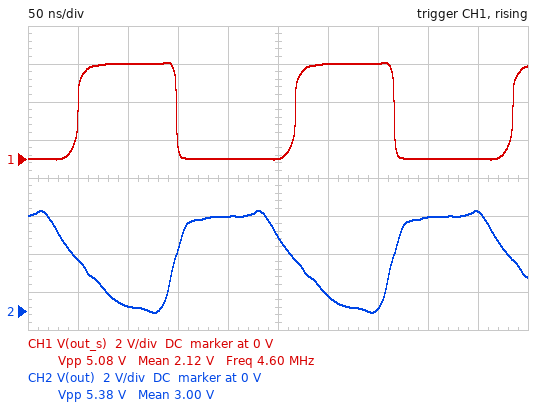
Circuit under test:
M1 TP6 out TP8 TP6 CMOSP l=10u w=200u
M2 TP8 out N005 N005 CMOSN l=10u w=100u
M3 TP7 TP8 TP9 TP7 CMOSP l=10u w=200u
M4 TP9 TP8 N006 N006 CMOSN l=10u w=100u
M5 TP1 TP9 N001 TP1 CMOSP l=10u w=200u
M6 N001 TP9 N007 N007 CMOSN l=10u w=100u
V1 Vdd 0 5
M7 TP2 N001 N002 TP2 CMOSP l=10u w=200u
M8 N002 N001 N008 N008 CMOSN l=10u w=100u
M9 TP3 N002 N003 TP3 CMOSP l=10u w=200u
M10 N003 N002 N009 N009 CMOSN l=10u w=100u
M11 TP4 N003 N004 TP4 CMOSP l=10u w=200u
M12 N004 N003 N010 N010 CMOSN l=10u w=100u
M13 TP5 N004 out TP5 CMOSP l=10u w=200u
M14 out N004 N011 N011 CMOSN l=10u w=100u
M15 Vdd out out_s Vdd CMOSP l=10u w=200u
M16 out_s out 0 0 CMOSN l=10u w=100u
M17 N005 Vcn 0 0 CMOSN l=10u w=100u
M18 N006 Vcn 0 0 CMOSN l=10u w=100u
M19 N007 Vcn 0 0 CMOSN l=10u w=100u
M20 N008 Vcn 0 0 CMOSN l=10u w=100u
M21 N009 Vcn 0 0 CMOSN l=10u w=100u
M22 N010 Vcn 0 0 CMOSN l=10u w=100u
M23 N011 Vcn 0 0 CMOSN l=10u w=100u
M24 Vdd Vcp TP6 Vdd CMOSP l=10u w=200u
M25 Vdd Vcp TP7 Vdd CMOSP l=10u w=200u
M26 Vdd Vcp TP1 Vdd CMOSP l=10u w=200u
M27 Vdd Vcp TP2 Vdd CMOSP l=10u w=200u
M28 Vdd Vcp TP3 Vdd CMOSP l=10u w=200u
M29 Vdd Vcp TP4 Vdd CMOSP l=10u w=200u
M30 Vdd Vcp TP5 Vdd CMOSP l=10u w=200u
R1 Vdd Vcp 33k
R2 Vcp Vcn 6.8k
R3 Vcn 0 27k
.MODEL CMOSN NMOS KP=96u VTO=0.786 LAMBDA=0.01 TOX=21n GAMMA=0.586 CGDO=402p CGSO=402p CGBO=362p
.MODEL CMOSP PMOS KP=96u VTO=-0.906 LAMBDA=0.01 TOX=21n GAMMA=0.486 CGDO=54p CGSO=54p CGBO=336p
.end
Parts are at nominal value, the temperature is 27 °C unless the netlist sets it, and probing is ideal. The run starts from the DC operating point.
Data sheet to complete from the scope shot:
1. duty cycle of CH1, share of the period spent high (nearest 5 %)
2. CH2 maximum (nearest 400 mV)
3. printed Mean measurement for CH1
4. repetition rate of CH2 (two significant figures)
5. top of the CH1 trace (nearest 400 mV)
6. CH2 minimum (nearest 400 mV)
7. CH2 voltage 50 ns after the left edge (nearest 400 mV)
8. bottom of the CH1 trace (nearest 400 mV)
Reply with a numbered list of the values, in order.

1. 45 %
2. 5.2 V
3. 2.12 V
4. 4.6 MHz
5. 5.2 V
6. 0 V
7. 2.8 V
8. 0 V
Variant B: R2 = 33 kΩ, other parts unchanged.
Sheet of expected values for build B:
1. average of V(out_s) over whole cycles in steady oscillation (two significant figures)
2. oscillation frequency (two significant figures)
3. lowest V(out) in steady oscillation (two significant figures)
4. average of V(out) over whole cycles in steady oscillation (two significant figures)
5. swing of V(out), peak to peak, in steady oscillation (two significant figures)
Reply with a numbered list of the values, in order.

1. 2.1 V
2. 1.6 MHz
3. -76 mV
4. 3.1 V
5. 5.2 V
